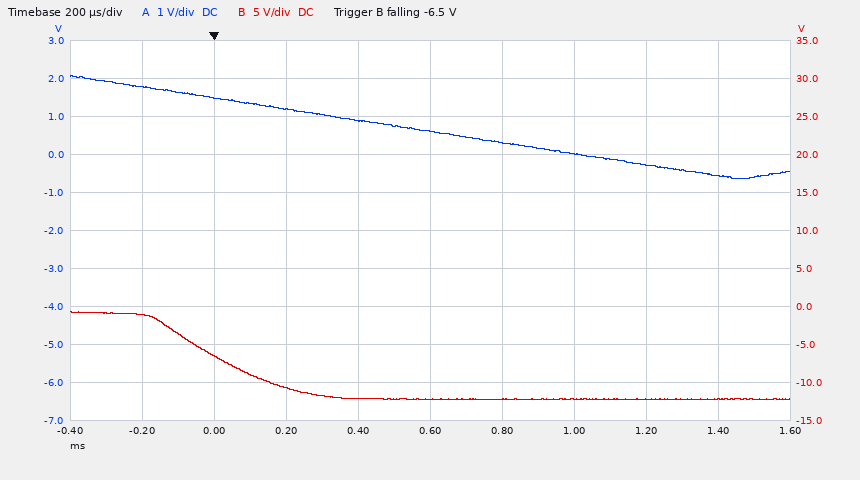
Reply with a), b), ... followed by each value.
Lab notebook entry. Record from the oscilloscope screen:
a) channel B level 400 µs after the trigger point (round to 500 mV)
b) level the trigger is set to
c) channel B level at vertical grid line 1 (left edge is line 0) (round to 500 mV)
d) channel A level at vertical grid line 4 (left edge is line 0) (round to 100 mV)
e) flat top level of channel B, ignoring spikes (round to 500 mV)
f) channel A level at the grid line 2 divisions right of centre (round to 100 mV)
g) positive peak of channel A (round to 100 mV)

a) -12.0 V
b) -6.5 V
c) -1.0 V
d) 900 mV
e) -1.0 V
f) 0.0 V
g) 2.1 V
